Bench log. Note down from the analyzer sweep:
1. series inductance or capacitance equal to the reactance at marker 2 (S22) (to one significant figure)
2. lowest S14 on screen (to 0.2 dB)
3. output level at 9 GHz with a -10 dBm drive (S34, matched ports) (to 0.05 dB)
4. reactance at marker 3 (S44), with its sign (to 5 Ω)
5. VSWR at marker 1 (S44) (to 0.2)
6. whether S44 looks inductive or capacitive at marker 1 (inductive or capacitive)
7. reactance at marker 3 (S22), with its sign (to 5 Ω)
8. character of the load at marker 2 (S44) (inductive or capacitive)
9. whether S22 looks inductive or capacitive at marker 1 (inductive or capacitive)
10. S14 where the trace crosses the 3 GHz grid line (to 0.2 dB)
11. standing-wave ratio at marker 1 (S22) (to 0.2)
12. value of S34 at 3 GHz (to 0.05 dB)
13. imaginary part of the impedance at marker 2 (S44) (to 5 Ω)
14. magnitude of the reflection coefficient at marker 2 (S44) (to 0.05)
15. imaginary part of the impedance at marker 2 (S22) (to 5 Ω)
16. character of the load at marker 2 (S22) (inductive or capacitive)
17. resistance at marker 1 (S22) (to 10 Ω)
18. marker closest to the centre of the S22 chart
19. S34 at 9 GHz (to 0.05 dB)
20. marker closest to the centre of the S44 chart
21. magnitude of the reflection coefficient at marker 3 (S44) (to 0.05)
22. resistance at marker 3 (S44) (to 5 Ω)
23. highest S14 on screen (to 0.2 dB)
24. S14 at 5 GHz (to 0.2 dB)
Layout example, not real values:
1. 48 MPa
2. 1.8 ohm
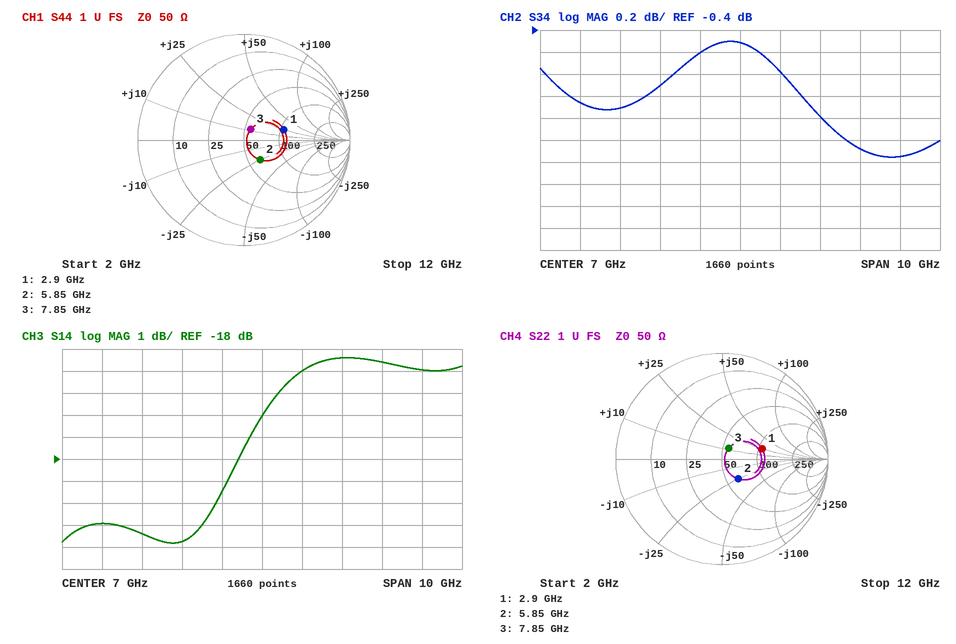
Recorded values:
1. 1 pF
2. -21.8 dB
3. -11.20 dBm
4. +10 Ω
5. 2.2
6. inductive
7. +10 Ω
8. capacitive
9. inductive
10. -21.0 dB
11. 2.2
12. -1.05 dB
13. -25 Ω
14. 0.25
15. -25 Ω
16. capacitive
17. 110 Ω
18. marker 3
19. -1.20 dB
20. marker 3
21. 0.10
22. 55 Ω
23. -13.4 dB
24. -21.8 dB
